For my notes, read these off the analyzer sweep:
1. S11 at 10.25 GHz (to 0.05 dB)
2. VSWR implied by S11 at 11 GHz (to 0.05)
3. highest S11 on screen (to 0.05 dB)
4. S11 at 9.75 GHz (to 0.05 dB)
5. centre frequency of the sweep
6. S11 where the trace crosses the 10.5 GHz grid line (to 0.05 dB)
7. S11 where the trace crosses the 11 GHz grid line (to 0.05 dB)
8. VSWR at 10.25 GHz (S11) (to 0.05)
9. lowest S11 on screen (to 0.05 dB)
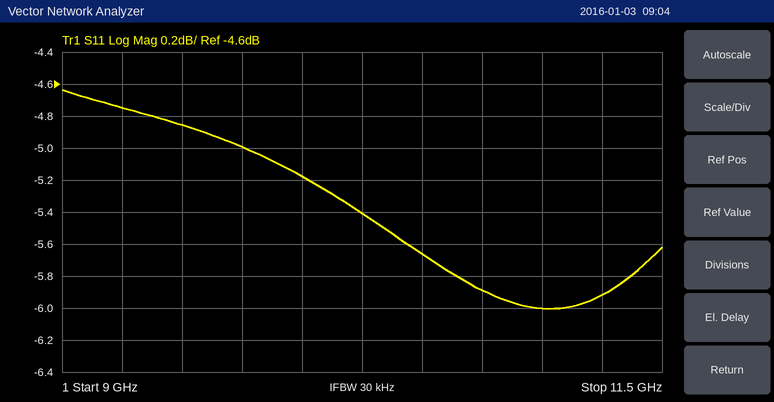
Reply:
-5.40 dB
3.00
-4.65 dB
-5.00 dB
10.25 GHz
-5.65 dB
-6.00 dB
3.30
-6.00 dB
